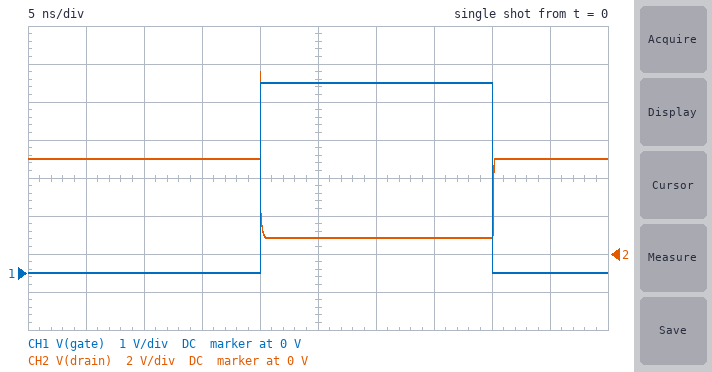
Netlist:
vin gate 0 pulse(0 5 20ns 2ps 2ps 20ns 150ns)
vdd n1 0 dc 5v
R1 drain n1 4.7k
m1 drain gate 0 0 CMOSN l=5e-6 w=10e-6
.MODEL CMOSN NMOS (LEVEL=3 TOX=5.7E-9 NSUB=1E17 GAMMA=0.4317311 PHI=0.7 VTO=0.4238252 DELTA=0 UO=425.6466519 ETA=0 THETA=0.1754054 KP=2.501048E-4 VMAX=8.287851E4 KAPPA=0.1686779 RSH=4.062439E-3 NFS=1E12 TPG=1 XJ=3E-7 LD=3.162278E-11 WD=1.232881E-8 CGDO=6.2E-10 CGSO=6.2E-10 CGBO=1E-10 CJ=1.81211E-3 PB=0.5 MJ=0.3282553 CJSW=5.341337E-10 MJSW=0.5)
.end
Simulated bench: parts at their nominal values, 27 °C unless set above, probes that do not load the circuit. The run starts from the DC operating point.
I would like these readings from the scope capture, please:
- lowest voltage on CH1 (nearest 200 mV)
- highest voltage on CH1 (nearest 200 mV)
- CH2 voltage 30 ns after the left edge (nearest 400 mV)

0 V
5.0 V
800 mV
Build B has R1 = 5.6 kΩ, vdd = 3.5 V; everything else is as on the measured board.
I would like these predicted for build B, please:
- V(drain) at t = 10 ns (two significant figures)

3.5 V
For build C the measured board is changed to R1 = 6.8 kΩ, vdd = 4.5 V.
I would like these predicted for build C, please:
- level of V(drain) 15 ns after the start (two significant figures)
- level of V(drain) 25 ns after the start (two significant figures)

4.5 V
510 mV
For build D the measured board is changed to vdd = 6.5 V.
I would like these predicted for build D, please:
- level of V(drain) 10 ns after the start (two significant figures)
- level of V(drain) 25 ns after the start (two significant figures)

6.5 V
1.1 V
